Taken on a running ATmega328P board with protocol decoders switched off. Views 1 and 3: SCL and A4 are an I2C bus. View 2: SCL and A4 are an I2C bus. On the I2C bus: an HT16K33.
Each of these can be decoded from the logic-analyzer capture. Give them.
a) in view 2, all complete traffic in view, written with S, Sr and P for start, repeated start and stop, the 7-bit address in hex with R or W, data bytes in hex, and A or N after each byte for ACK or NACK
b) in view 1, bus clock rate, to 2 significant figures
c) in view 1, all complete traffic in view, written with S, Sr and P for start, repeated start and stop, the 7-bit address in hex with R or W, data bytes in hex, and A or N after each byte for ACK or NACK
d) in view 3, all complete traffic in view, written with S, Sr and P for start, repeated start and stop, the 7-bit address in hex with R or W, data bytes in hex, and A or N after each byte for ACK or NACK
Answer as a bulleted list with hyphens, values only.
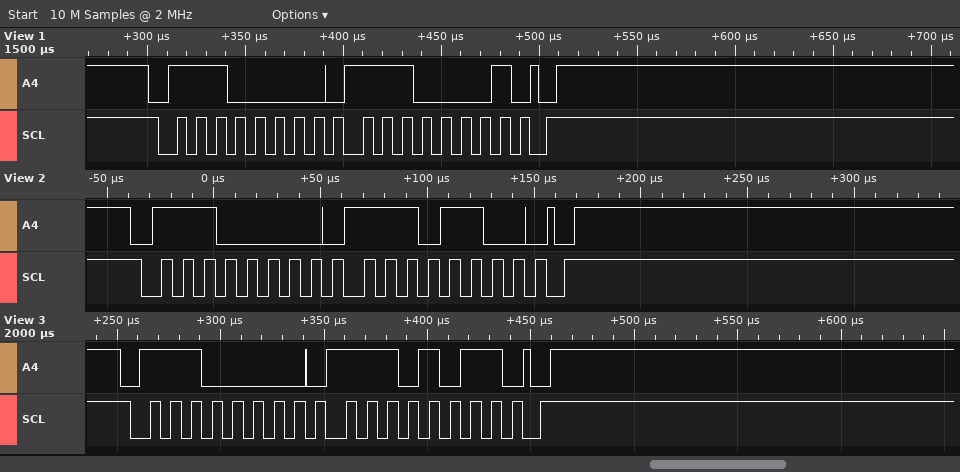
- S 70W A EC A P
- 100 kHz
- S 70W A E1 A P
- S 70W A EB A P
